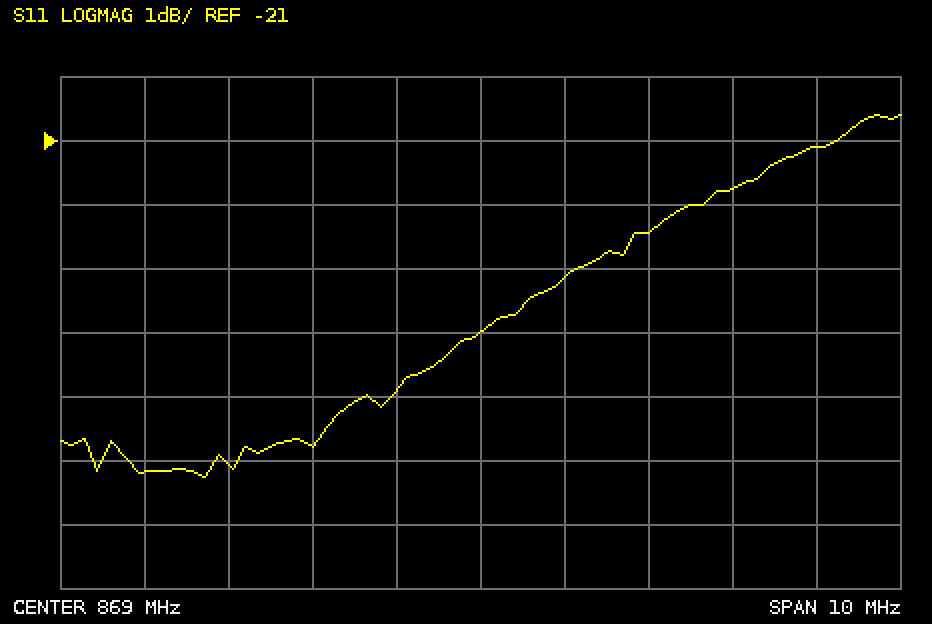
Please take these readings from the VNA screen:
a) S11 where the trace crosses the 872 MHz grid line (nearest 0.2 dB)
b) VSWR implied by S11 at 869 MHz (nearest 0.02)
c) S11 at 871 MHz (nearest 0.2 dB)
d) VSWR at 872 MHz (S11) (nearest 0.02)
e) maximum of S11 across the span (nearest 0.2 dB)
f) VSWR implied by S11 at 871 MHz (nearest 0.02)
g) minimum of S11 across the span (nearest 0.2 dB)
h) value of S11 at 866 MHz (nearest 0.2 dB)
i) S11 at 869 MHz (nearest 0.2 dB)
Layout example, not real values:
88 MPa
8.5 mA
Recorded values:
-21.8 dB
1.14
-22.4 dB
1.18
-20.6 dB
1.16
-26.2 dB
-26.0 dB
-24.0 dB
